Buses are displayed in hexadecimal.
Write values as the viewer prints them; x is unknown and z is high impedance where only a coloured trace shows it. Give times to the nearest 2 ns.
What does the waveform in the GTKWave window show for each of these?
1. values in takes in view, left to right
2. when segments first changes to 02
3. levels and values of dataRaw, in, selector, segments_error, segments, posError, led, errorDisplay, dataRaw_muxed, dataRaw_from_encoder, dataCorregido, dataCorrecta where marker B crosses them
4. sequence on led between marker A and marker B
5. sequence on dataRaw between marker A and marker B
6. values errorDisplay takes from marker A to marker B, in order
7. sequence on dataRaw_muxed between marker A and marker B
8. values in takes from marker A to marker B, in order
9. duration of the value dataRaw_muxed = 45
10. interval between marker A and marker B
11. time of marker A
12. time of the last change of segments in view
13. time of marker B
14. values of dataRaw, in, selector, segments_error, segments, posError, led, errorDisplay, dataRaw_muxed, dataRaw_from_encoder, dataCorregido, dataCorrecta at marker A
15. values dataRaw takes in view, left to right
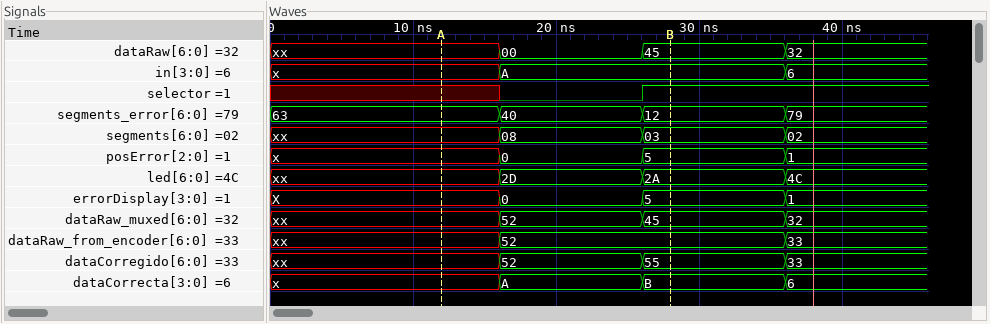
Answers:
x, A, 6
36 ns
dataRaw=45, in=A, selector=1, segments_error=12, segments=03, posError=5, led=2A, errorDisplay=5, dataRaw_muxed=45, dataRaw_from_encoder=52, dataCorregido=55, dataCorrecta=B
xx, 2D, 2A
xx, 00, 45
X, 0, 5
xx, 52, 45
x, A
10 ns
16 ns
12 ns
36 ns
28 ns
dataRaw=xx, in=x, selector=x, segments_error=63, segments=xx, posError=x, led=xx, errorDisplay=X, dataRaw_muxed=xx, dataRaw_from_encoder=xx, dataCorregido=xx, dataCorrecta=x
xx, 00, 45, 32
